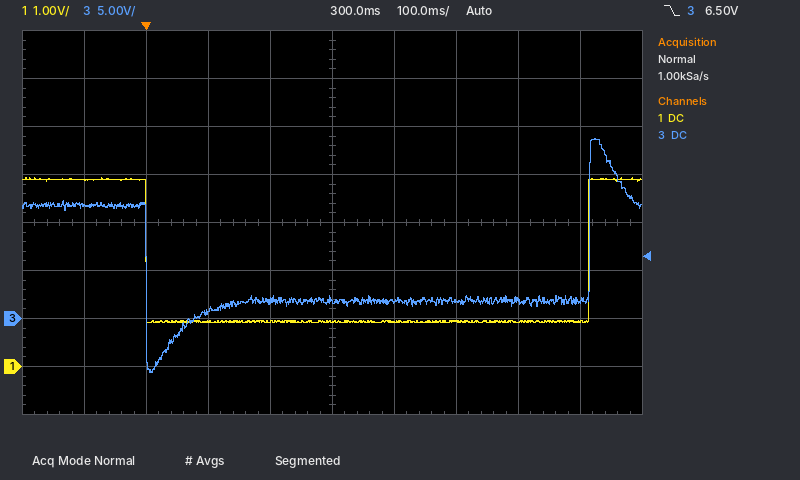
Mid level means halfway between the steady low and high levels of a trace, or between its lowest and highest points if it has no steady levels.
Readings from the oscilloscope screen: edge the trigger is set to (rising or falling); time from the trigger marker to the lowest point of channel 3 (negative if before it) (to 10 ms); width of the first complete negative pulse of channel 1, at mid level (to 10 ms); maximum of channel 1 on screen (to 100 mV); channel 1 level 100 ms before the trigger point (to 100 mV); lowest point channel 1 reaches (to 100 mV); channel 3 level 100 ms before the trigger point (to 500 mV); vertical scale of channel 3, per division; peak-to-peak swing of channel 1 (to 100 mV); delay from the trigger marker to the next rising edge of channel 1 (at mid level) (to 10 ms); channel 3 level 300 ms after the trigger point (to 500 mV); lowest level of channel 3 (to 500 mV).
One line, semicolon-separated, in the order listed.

falling; +10 ms; 710 ms; 3.9 V; 3.9 V; 900 mV; 12.0 V; 5 V; 3.0 V; 710 ms; 2.0 V; -5.5 V
